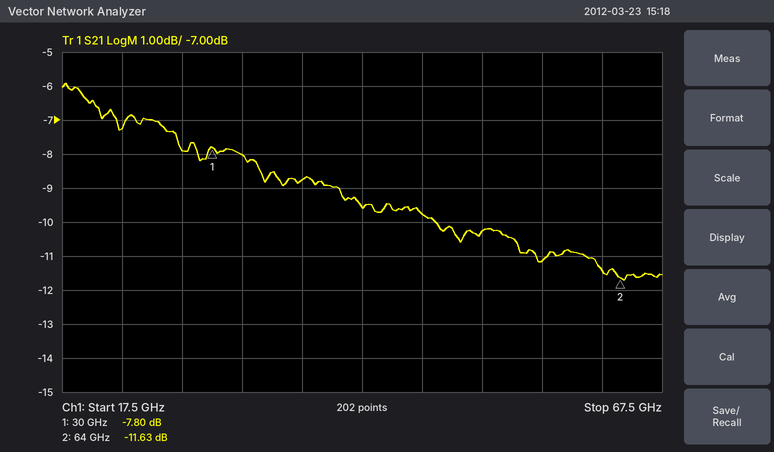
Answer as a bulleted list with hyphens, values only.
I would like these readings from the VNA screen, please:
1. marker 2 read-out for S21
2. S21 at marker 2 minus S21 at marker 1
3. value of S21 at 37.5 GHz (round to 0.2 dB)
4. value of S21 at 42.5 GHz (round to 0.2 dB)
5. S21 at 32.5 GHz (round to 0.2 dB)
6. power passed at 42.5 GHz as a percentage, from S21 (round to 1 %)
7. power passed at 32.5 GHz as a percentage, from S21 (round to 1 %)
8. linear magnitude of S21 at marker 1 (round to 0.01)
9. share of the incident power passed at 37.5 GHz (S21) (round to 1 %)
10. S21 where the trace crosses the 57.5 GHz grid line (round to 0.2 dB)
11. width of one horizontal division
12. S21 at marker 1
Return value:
- -11.63 dB
- -3.83 dB
- -8.8 dB
- -9.6 dB
- -8.0 dB
- 11 %
- 16 %
- 0.41
- 13 %
- -11.2 dB
- 5 GHz
- -7.80 dB
